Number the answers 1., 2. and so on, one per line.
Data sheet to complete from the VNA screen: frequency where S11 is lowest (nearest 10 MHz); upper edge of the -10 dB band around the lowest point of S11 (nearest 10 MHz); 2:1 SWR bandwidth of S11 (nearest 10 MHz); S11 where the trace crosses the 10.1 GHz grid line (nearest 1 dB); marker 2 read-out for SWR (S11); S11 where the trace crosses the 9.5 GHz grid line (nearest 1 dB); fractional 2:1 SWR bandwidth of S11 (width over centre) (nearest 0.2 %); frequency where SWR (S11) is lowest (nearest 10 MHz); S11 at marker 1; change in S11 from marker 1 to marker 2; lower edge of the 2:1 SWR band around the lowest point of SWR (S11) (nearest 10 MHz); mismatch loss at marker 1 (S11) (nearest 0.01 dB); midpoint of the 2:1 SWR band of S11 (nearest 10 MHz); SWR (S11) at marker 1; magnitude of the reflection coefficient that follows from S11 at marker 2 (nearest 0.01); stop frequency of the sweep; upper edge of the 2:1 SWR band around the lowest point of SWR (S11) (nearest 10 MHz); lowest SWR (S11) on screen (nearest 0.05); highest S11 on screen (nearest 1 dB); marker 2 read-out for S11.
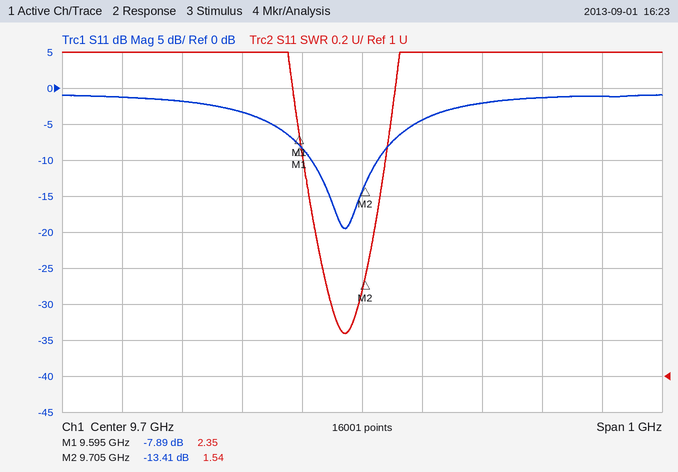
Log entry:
1. 9.67 GHz
2. 9.73 GHz
3. 120 MHz
4. -1 dB
5. 1.54
6. -3 dB
7. 1.2 %
8. 9.67 GHz
9. -7.89 dB
10. -5.52 dB
11. 9.61 GHz
12. 0.77 dB
13. 9.67 GHz
14. 2.35
15. 0.21
16. 10.2 GHz
17. 9.73 GHz
18. 1.25
19. -1 dB
20. -13.41 dB
